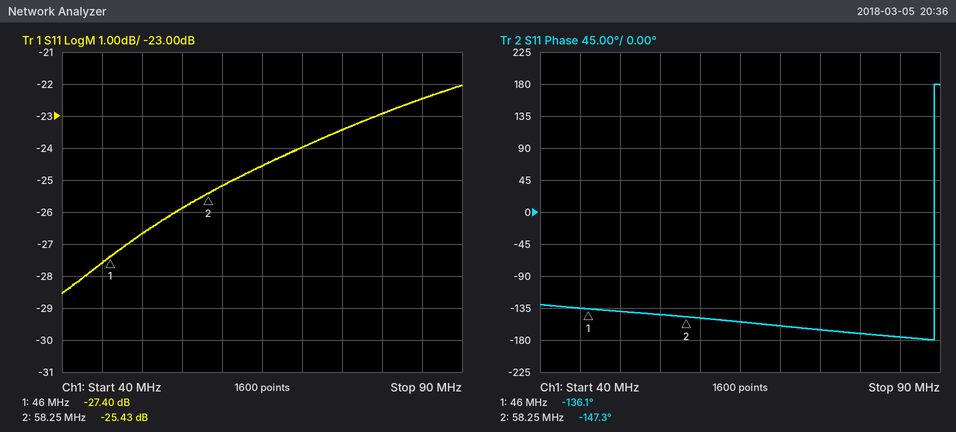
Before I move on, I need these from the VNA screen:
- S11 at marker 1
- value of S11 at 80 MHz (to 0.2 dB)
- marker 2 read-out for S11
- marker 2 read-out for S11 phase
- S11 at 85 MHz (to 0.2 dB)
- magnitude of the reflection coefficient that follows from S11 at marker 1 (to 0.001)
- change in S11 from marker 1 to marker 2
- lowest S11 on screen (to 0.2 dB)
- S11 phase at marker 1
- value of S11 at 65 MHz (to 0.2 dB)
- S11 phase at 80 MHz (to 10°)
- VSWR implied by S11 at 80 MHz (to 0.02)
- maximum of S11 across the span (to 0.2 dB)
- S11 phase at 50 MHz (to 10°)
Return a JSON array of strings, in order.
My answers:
["-27.40 dB", "-23.0 dB", "-25.43 dB", "-147.3°", "-22.4 dB", "0.043", "1.97 dB", "-28.6 dB", "-136.1°", "-24.6 dB", "-170°", "1.16", "-22.0 dB", "-140°"]
